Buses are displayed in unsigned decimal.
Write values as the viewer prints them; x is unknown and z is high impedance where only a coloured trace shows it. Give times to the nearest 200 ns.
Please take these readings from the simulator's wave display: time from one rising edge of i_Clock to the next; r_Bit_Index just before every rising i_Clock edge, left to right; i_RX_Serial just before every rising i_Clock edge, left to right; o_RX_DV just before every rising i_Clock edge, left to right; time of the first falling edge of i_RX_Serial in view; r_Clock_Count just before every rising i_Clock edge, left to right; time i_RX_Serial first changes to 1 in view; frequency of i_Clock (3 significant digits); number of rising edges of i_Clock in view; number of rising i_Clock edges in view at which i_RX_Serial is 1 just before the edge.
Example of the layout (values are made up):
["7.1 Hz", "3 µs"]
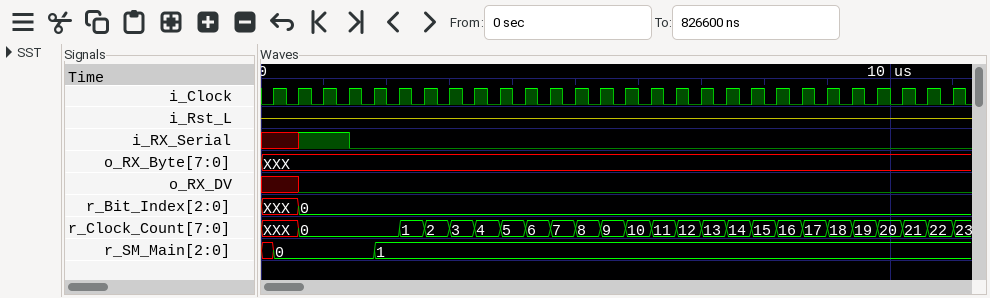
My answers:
["400 ns", "XXX, XXX, 0, 0, 0, 0, 0, 0, 0, 0, 0, 0, 0, 0, 0, 0, 0, 0, 0, 0, 0, 0, 0, 0, 0, 0, 0, 0", "x x 1 1 0 0 0 0 0 0 0 0 0 0 0 0 0 0 0 0 0 0 0 0 0 0 0 0", "x x 0 0 0 0 0 0 0 0 0 0 0 0 0 0 0 0 0 0 0 0 0 0 0 0 0 0", "1400 ns", "XXX, XXX, 0, 0, 0, 0, 1, 2, 3, 4, 5, 6, 7, 8, 9, 10, 11, 12, 13, 14, 15, 16, 17, 18, 19, 20, 21, 22", "600 ns", "2.50 MHz", "28", "2"]
